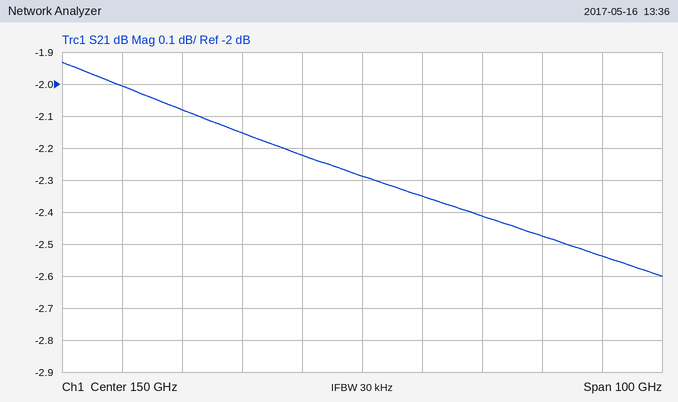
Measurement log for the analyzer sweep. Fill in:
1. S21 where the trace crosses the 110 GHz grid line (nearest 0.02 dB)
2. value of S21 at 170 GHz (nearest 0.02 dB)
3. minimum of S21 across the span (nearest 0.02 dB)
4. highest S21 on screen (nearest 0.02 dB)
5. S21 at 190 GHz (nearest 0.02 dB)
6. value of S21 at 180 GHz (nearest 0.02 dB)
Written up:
-2.00 dB
-2.42 dB
-2.60 dB
-1.94 dB
-2.54 dB
-2.48 dB
